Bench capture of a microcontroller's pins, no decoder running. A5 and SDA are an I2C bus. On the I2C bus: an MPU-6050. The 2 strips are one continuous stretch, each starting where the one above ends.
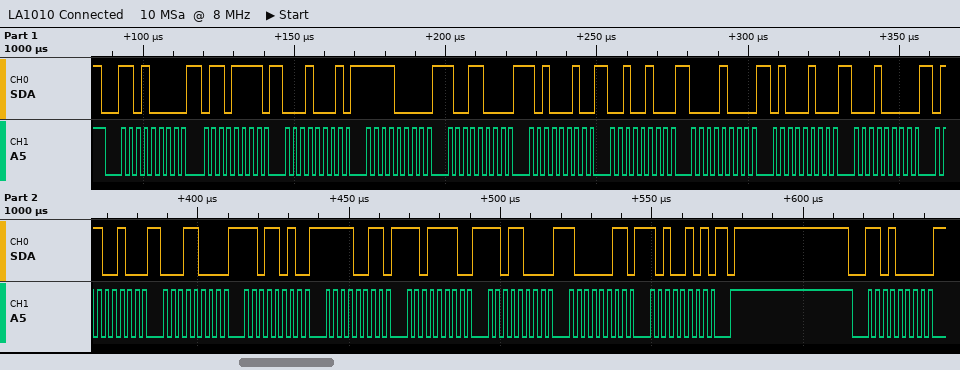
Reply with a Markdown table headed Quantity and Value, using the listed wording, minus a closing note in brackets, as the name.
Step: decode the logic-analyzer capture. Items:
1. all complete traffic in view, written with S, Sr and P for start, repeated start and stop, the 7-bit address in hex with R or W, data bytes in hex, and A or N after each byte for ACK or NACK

| Quantity | Value |
|---|---|
| all complete traffic in view, written with S, Sr and P for start, repeated start and stop, the 7-bit address in hex with R or W, data bytes in hex, and A or N after each byte for ACK or NACK | S 68W A 6F A 11 A F0 A 98 A A2 A 24 A 08 A 44 A 10 A 64 A 18 A DA A F3 A DE A D8 A 83 A A5 A P S 68W A |
